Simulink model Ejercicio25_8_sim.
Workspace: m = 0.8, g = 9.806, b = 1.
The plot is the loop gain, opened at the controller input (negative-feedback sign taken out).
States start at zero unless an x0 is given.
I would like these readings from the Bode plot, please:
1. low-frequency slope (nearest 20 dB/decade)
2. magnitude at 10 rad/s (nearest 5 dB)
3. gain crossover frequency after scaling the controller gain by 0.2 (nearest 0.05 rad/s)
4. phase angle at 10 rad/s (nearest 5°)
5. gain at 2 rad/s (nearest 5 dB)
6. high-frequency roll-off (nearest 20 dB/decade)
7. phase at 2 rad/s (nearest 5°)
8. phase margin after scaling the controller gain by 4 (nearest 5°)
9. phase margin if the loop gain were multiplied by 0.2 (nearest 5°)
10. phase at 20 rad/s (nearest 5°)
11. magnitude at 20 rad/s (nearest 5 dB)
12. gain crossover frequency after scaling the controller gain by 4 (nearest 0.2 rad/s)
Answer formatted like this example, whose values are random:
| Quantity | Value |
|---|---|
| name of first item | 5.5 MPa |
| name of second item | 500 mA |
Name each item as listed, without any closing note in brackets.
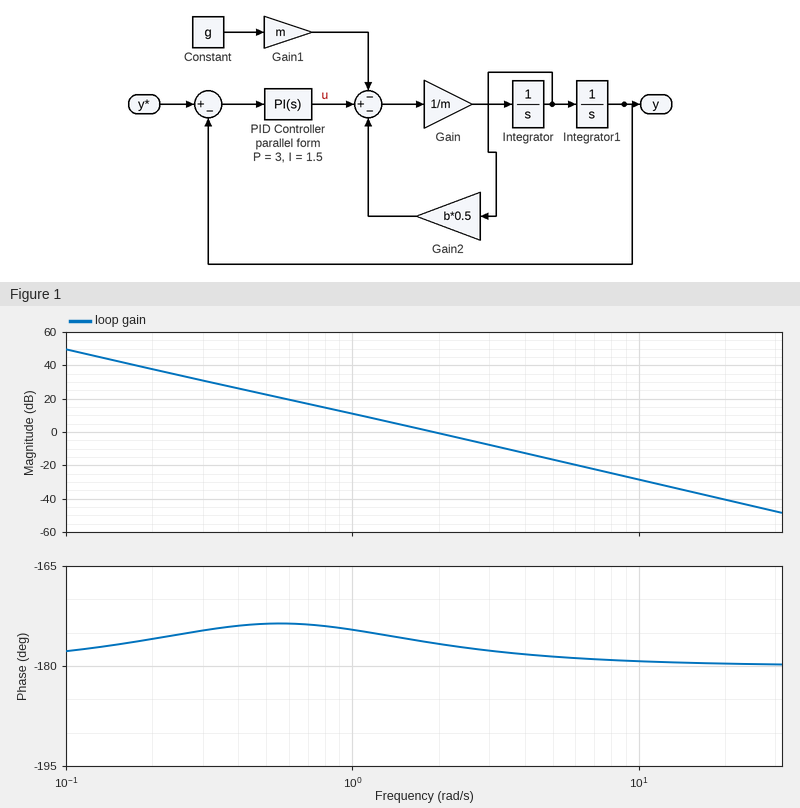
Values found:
| Quantity | Value |
|---|---|
| low-frequency slope | -40 dB/decade |
| magnitude at 10 rad/s | -30 dB |
| gain crossover frequency after scaling the controller gain by 0.2 | 0.85 rad/s |
| phase angle at 10 rad/s | -180° |
| gain at 2 rad/s | 0 dB |
| high-frequency roll-off | -40 dB/decade |
| phase at 2 rad/s | -175° |
| phase margin after scaling the controller gain by 4 | 0° |
| phase margin if the loop gain were multiplied by 0.2 | 5° |
| phase at 20 rad/s | -180° |
| magnitude at 20 rad/s | -40 dB |
| gain crossover frequency after scaling the controller gain by 4 | 3.8 rad/s |
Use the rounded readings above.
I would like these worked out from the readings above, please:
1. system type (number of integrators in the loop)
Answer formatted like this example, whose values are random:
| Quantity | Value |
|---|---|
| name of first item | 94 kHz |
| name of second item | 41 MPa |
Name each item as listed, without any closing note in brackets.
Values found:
| Quantity | Value |
|---|---|
| system type | 2 |
